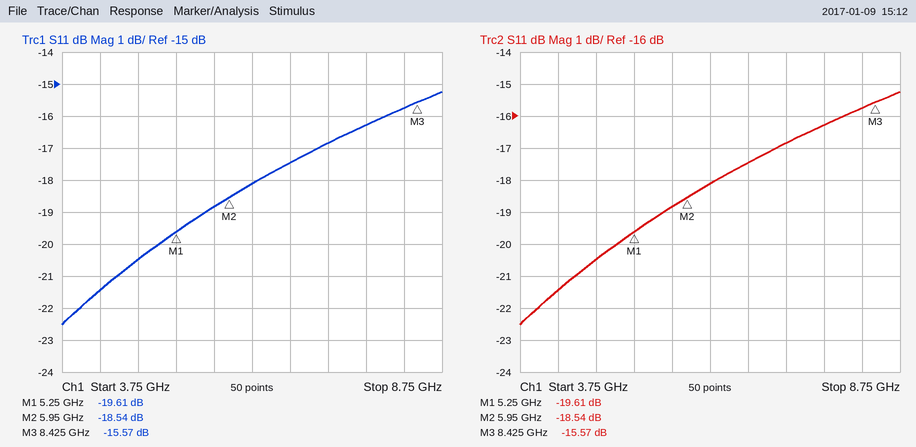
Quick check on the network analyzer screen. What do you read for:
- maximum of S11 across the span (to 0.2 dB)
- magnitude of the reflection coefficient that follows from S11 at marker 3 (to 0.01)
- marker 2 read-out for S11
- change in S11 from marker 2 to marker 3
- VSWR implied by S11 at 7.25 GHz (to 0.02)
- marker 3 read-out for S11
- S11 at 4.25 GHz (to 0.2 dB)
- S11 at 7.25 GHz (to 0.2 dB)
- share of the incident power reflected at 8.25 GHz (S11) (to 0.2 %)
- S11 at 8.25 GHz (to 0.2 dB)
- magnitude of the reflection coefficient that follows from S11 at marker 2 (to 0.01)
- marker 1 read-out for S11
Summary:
-15.2 dB
0.17
-18.54 dB
2.97 dB
1.34
-15.57 dB
-21.4 dB
-16.8 dB
2.6 %
-15.8 dB
0.12
-19.61 dB
